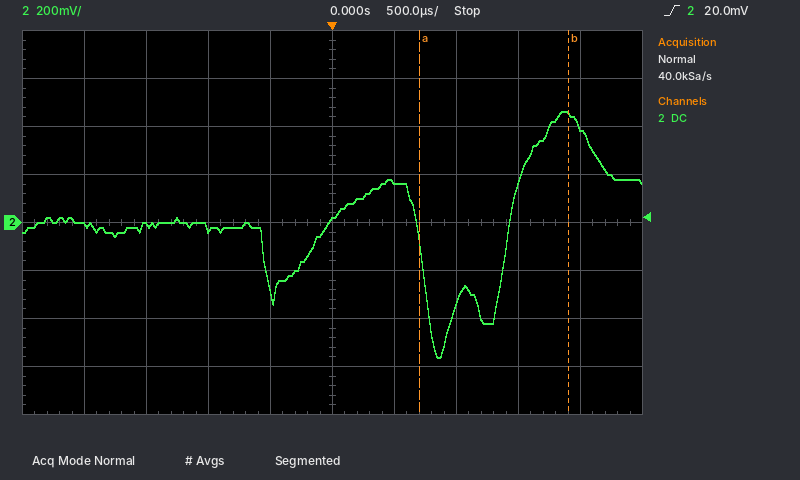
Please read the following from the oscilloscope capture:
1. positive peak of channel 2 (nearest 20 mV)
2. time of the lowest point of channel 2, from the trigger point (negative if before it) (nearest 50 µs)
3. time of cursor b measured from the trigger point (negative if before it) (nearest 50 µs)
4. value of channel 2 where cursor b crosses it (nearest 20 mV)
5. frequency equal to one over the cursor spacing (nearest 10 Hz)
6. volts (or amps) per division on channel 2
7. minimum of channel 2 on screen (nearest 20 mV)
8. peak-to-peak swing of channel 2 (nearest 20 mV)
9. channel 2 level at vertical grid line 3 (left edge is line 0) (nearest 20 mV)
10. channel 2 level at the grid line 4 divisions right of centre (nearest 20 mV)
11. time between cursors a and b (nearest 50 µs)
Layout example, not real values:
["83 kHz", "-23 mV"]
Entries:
["460 mV", "+850 µs", "+1.90 ms", "460 mV", "830 Hz", "200 mV", "-560 mV", "1.02 V", "-20 mV", "400 mV", "1.20 ms"]
